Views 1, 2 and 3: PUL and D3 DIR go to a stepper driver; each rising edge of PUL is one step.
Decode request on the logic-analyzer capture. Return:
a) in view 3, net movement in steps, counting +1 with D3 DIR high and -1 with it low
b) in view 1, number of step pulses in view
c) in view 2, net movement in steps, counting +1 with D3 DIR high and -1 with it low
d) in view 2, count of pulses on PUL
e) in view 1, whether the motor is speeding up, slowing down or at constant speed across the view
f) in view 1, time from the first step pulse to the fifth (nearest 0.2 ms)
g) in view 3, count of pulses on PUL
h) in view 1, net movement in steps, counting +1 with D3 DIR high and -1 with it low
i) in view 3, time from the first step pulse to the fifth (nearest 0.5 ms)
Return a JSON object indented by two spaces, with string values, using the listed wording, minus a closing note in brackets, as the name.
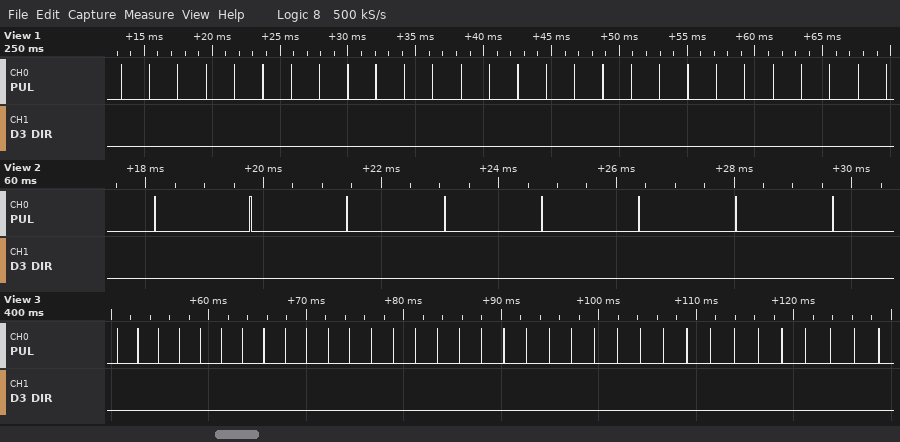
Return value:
{
  "in view 3, net movement in steps, counting +1 with D3 DIR high and -1 with it low": "-35",
  "in view 1, number of step pulses in view": "28",
  "in view 2, net movement in steps, counting +1 with D3 DIR high and -1 with it low": "-8",
  "in view 2, count of pulses on PUL": "8",
  "in view 1, whether the motor is speeding up, slowing down or at constant speed across the view": "constant speed",
  "in view 1, time from the first step pulse to the fifth": "8.4 ms",
  "in view 3, count of pulses on PUL": "35",
  "in view 1, net movement in steps, counting +1 with D3 DIR high and -1 with it low": "-28",
  "in view 3, time from the first step pulse to the fifth": "8.5 ms"
}
